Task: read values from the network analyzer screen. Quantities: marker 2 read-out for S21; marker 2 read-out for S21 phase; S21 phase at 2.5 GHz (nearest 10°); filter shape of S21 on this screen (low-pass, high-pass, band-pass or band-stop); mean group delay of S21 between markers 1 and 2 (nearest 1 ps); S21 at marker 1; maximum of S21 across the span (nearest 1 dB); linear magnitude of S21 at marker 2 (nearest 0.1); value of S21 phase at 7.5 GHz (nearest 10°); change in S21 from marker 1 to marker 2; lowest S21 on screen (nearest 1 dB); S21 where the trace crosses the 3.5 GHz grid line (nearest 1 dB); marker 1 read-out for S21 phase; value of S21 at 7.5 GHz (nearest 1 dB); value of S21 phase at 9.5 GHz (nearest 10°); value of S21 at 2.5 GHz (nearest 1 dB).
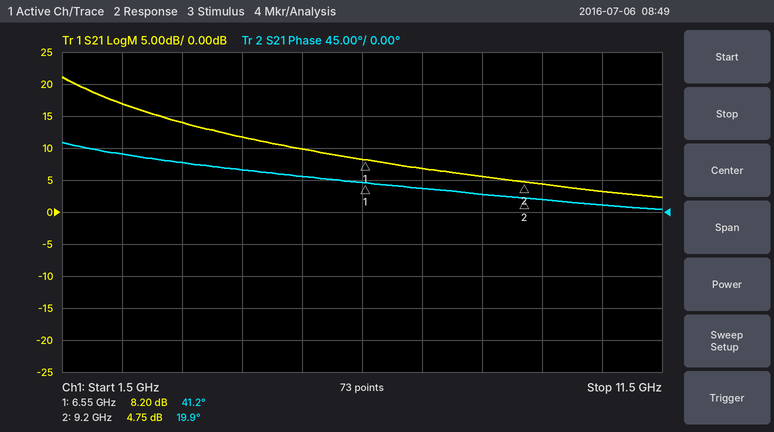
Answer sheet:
4.75 dB
19.9°
80°
low-pass
22 ps
8.20 dB
21 dB
1.7
30°
-3.45 dB
2 dB
14 dB
41.2°
7 dB
20°
17 dB
